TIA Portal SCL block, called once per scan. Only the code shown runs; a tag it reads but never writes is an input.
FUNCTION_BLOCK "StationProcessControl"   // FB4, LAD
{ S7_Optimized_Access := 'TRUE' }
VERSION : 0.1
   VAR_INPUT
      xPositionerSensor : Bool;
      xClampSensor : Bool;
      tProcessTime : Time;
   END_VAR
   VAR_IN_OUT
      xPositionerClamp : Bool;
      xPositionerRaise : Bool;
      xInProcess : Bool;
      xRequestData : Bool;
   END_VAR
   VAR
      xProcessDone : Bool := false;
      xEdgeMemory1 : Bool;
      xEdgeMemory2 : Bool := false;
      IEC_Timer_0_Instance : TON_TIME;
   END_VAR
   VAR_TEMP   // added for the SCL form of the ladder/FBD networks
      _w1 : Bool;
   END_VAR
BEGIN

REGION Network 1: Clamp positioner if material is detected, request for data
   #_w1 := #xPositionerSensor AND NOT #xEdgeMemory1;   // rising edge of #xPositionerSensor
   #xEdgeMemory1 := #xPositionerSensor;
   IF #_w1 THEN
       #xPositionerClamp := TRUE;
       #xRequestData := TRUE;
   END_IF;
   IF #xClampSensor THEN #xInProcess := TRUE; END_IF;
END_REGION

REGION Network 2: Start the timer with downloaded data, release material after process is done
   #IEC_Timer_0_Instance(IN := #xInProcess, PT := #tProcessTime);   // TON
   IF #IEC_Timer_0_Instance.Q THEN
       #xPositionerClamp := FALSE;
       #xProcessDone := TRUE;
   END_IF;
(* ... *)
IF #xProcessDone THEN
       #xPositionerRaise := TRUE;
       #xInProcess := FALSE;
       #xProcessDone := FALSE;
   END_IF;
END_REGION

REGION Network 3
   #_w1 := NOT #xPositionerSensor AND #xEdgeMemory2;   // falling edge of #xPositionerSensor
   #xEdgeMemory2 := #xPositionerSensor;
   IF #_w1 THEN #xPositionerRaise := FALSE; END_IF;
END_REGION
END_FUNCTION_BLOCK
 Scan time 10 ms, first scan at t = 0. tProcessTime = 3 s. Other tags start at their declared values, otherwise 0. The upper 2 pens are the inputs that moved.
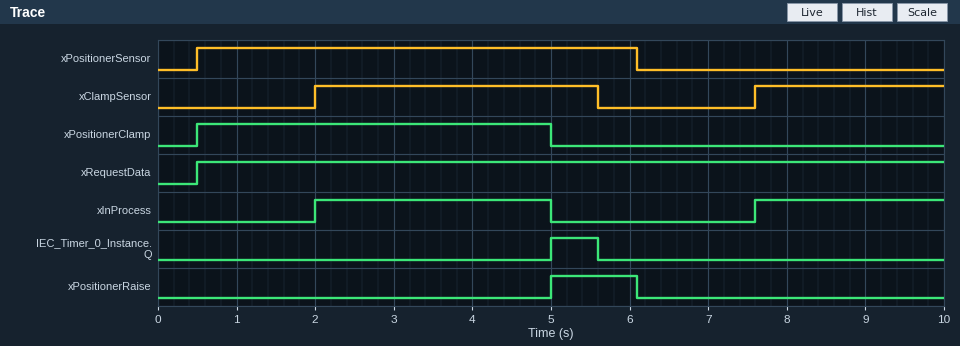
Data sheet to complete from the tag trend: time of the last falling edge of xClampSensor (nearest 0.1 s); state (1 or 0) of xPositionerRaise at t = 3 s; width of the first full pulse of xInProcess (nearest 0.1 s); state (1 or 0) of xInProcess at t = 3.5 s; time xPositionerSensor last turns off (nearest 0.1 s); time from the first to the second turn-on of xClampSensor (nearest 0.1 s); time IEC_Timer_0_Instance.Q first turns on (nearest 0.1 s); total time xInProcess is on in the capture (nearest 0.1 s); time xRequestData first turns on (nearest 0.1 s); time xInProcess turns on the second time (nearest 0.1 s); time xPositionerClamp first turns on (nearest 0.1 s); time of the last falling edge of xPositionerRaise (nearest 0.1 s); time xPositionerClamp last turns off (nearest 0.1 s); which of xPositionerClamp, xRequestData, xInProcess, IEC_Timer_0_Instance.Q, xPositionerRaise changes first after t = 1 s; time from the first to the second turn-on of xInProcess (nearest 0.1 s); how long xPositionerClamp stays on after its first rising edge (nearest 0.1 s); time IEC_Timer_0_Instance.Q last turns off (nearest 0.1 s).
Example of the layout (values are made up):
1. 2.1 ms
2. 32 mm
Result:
1. 5.6 s
2. 0
3. 3.0 s
4. 1
5. 6.1 s
6. 5.6 s
7. 5.0 s
8. 5.4 s
9. 0.5 s
10. 7.6 s
11. 0.5 s
12. 6.1 s
13. 5.0 s
14. xInProcess
15. 5.6 s
16. 4.5 s
17. 5.6 s
